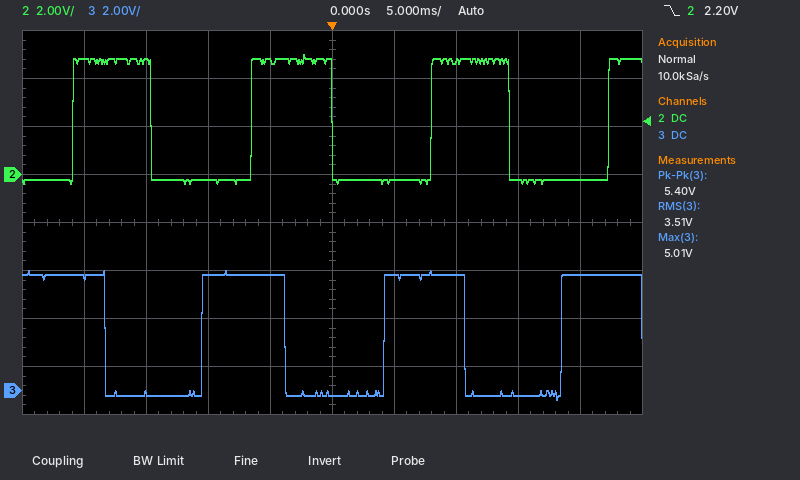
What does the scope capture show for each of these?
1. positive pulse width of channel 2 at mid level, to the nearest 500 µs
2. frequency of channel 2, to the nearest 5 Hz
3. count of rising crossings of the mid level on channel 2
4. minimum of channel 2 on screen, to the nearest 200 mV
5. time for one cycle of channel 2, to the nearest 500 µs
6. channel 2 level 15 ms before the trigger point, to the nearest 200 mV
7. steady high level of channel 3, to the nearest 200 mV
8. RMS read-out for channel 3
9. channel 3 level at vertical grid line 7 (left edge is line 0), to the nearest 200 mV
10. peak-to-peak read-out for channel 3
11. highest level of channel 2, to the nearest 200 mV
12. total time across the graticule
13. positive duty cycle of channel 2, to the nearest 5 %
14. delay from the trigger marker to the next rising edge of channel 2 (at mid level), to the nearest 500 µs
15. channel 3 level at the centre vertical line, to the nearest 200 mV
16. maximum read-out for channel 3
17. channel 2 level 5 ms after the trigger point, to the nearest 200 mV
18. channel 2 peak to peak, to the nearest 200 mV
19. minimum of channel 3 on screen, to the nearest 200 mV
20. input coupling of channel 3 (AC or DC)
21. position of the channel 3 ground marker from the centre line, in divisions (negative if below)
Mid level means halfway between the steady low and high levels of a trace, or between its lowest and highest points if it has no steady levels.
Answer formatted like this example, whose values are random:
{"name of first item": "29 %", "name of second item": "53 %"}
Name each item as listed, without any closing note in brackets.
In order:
{"positive pulse width of channel 2 at mid level, to the nearest 500 µs": "6.5 ms", "frequency of channel 2, to the nearest 5 Hz": "70 Hz", "count of rising crossings of the mid level on channel 2": "4", "minimum of channel 2 on screen, to the nearest 200 mV": "-400 mV", "time for one cycle of channel 2, to the nearest 500 µs": "14.5 ms", "channel 2 level 15 ms before the trigger point, to the nearest 200 mV": "4.8 V", "steady high level of channel 3, to the nearest 200 mV": "4.8 V", "RMS read-out for channel 3": "3.51 V", "channel 3 level at vertical grid line 7 (left edge is line 0), to the nearest 200 mV": "4.8 V", "peak-to-peak read-out for channel 3": "5.40 V", "highest level of channel 2, to the nearest 200 mV": "5.0 V", "total time across the graticule": "50 ms", "positive duty cycle of channel 2, to the nearest 5 %": "45 %", "delay from the trigger marker to the next rising edge of channel 2 (at mid level), to the nearest 500 µs": "8.0 ms", "channel 3 level at the centre vertical line, to the nearest 200 mV": "-200 mV", "maximum read-out for channel 3": "5.01 V", "channel 2 level 5 ms after the trigger point, to the nearest 200 mV": "-200 mV", "channel 2 peak to peak, to the nearest 200 mV": "5.4 V", "minimum of channel 3 on screen, to the nearest 200 mV": "-400 mV", "input coupling of channel 3": "DC", "position of the channel 3 ground marker from the centre line, in divisions": "-3.5 div"}
